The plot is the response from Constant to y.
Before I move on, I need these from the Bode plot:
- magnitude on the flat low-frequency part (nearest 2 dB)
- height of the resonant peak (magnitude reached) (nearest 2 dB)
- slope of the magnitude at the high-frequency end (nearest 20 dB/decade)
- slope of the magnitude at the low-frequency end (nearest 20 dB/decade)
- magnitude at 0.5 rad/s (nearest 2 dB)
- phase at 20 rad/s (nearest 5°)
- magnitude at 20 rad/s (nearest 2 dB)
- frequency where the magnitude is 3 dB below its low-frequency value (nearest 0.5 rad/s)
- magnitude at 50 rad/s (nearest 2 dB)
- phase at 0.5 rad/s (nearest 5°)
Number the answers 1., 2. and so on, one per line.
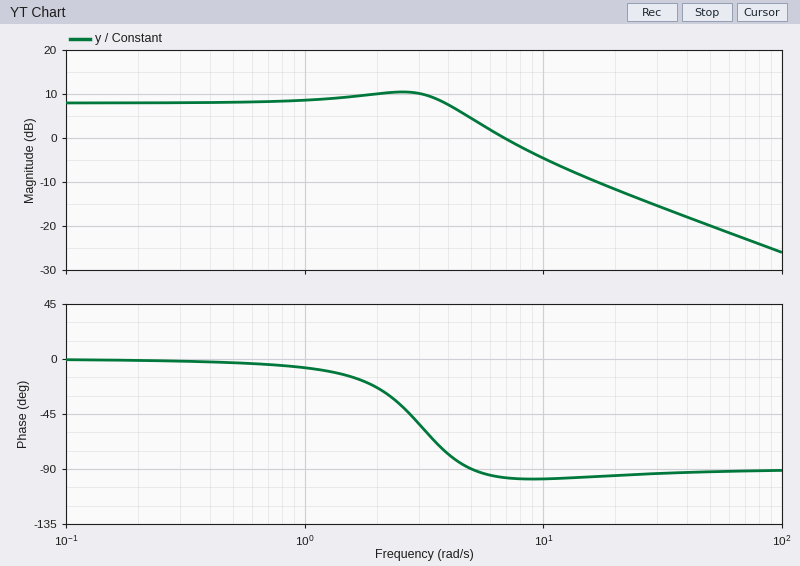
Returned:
1. 8 dB
2. 10 dB
3. -20 dB/decade
4. 0 dB/decade
5. 8 dB
6. -95°
7. -12 dB
8. 5.0 rad/s
9. -20 dB
10. -5°
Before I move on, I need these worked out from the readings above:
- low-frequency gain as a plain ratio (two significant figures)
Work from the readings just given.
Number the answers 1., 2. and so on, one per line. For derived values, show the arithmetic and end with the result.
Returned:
1. 10^(8 / 20) = 2.5
